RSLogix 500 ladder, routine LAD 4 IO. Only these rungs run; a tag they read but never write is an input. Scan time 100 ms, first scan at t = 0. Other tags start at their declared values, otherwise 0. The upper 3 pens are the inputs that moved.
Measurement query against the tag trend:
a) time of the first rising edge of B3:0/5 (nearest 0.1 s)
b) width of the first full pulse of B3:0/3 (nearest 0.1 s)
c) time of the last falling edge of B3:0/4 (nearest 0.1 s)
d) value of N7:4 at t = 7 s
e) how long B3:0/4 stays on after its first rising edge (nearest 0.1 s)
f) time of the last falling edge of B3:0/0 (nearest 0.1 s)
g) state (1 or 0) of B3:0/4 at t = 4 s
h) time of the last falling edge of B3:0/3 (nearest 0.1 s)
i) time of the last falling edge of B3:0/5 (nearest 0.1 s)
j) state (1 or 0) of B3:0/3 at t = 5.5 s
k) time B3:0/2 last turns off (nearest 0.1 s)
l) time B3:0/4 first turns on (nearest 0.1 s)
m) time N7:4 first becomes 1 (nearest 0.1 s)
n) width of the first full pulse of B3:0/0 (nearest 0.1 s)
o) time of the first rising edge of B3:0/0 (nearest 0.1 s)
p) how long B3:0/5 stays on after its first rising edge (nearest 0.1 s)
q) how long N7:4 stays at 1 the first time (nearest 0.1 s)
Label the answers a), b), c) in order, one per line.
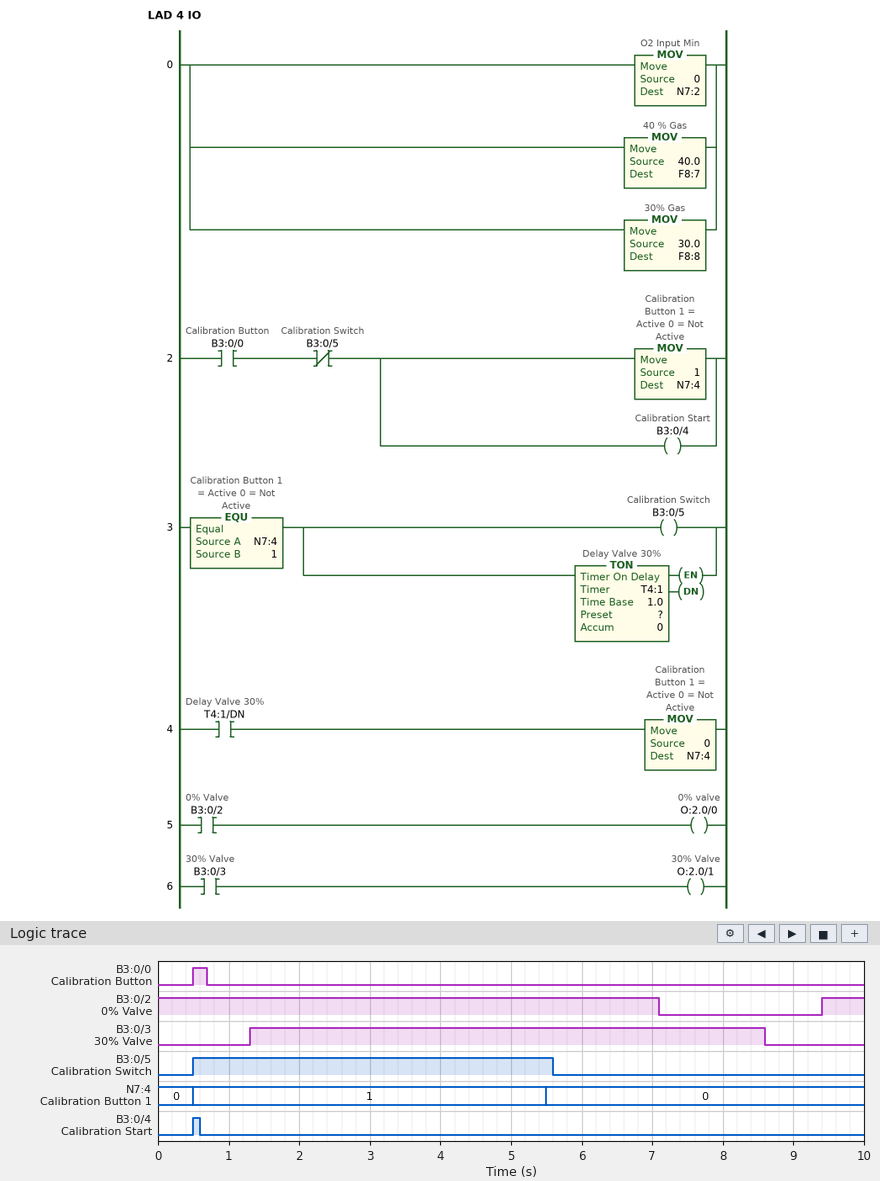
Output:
a) 0.5 s
b) 7.3 s
c) 0.6 s
d) 0
e) 0.1 s
f) 0.7 s
g) 0
h) 8.6 s
i) 5.6 s
j) 1
k) 7.1 s
l) 0.5 s
m) 0.5 s
n) 0.2 s
o) 0.5 s
p) 5.1 s
q) 5.0 s
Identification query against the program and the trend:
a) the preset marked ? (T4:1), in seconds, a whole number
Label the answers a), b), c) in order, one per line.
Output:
a) 5 s
